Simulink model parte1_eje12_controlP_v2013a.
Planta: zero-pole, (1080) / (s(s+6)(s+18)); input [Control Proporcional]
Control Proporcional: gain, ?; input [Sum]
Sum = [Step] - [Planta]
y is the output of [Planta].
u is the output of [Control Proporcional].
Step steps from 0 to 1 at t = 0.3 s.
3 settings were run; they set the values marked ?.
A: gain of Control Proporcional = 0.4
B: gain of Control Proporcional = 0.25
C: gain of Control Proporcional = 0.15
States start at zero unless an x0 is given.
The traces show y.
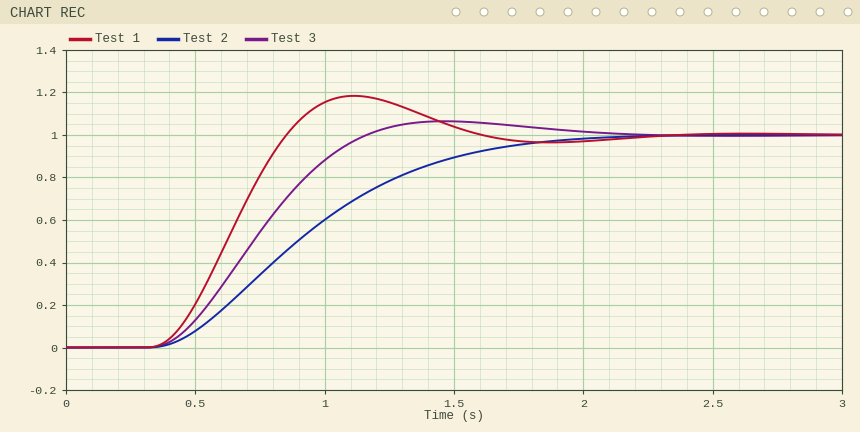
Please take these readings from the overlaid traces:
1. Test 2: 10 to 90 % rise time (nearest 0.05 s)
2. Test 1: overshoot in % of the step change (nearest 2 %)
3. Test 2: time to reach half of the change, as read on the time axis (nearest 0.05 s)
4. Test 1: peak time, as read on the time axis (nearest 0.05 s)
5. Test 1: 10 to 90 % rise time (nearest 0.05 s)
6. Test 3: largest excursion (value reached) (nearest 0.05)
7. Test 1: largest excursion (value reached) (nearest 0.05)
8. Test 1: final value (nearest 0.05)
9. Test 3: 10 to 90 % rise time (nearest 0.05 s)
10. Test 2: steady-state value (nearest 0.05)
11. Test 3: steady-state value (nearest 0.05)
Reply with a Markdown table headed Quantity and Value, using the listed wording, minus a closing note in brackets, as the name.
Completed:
| Quantity | Value |
|---|---|
| Test 2: 10 to 90 % rise time | 1.00 s |
| Test 1: overshoot in % of the step change | 18 % |
| Test 2: time to reach half of the change, as read on the time axis | 0.90 s |
| Test 1: peak time, as read on the time axis | 1.10 s |
| Test 1: 10 to 90 % rise time | 0.35 s |
| Test 3: largest excursion (value reached) | 1.05 |
| Test 1: largest excursion (value reached) | 1.20 |
| Test 1: final value | 1.00 |
| Test 3: 10 to 90 % rise time | 0.55 s |
| Test 2: steady-state value | 1.00 |
| Test 3: steady-state value | 1.00 |
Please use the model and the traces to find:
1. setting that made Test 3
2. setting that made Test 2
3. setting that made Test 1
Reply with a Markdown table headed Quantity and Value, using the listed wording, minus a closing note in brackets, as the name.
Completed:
| Quantity | Value |
|---|---|
| setting that made Test 3 | B |
| setting that made Test 2 | C |
| setting that made Test 1 | A |
